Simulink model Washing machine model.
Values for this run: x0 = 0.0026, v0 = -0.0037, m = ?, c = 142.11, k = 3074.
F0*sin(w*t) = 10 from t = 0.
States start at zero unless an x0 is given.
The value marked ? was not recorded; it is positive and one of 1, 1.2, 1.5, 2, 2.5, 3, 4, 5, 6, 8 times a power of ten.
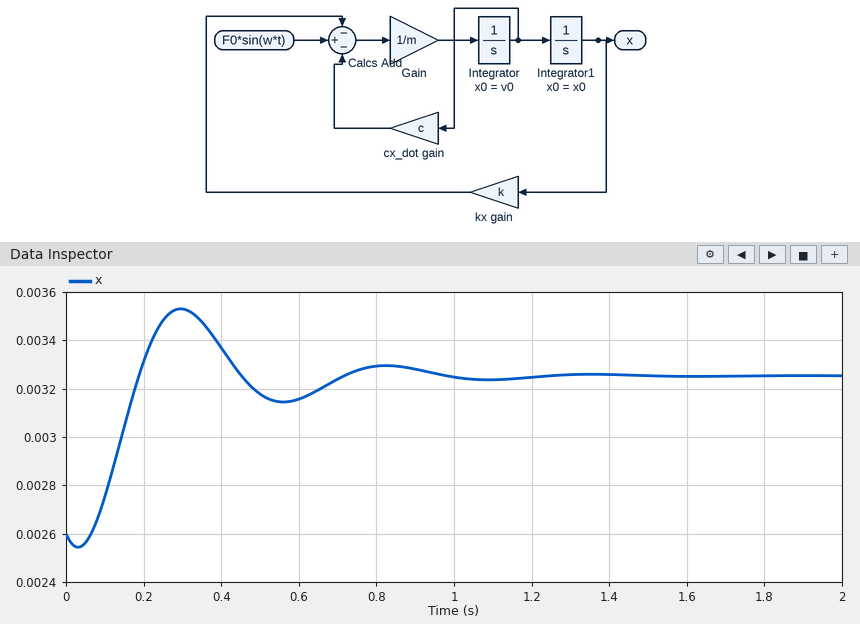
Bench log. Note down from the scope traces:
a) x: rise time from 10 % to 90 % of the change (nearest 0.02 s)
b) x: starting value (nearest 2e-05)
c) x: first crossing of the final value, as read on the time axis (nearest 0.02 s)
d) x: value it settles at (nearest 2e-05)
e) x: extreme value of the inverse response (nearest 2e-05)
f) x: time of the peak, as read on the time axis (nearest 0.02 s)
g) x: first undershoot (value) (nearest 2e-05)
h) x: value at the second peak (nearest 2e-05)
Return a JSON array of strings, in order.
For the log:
["0.10 s", "0.00260", "0.18 s", "0.00326", "0.00254", "0.30 s", "0.00314", "0.00330"]
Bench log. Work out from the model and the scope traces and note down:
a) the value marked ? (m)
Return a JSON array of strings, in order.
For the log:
["20"]
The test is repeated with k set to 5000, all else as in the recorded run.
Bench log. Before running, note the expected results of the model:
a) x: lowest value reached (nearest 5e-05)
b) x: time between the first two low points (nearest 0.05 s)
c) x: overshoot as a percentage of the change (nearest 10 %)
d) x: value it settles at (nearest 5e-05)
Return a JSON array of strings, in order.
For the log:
["0.00170", "0.40 s", "50 %", "0.00200"]
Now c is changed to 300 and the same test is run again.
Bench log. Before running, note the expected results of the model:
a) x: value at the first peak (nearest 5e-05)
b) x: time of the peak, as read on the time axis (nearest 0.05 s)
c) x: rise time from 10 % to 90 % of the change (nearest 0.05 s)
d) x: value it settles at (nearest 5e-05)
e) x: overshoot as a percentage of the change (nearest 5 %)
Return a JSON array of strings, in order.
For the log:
["0.00330", "0.35 s", "0.15 s", "0.00325", "10 %"]
